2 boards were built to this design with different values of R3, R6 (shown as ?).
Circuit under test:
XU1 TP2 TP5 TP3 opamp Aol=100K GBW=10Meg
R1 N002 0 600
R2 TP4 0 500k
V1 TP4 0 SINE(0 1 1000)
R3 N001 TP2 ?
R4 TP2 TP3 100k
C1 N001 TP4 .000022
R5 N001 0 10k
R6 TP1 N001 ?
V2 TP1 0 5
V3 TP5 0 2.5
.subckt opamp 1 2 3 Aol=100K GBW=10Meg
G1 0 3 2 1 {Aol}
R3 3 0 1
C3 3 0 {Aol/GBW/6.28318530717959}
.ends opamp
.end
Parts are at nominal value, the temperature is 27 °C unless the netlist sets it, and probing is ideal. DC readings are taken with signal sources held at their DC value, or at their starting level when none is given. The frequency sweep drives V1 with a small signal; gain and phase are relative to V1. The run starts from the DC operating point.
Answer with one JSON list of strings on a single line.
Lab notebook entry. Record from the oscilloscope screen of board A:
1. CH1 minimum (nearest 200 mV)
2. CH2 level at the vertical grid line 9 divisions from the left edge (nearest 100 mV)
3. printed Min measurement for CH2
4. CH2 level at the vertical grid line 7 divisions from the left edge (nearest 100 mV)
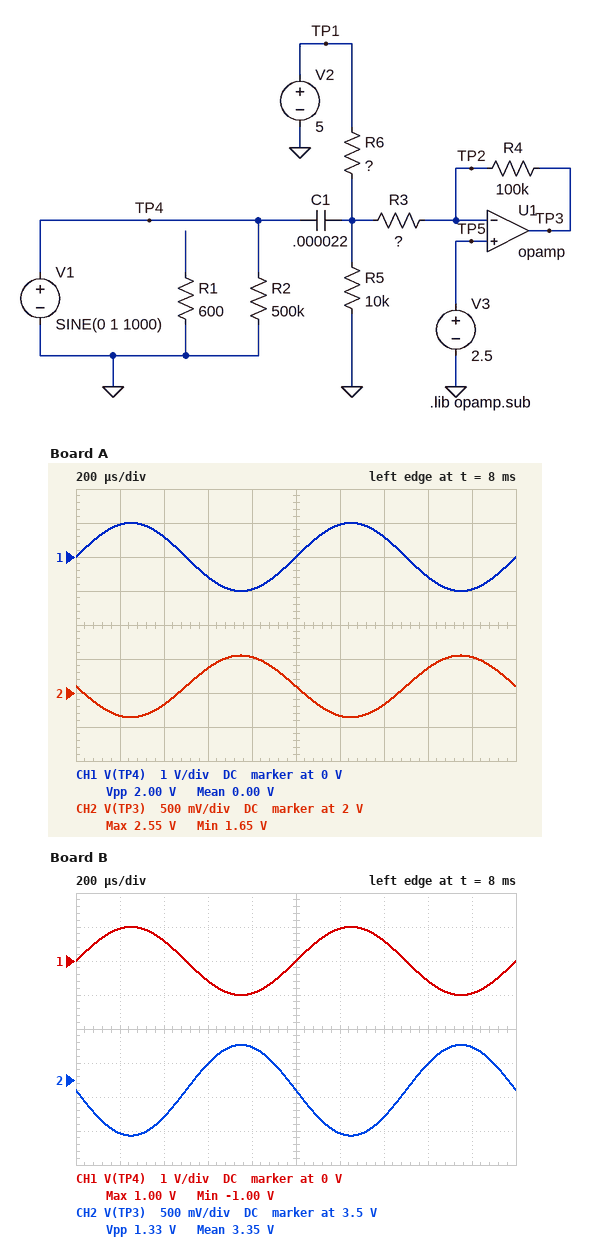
["-1.0 V", "2.5 V", "1.65 V", "1.8 V"]
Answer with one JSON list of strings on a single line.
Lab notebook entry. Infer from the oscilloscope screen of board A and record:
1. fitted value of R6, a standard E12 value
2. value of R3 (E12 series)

["4.7 kΩ", "220 kΩ"]
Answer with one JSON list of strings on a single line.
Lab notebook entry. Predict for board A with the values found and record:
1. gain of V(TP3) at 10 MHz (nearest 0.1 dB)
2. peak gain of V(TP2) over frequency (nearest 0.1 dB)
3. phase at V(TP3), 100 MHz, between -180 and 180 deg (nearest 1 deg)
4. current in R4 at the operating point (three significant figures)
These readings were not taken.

["-11.8 dB", "-10.1 dB", "94 deg", "4.04 µA"]
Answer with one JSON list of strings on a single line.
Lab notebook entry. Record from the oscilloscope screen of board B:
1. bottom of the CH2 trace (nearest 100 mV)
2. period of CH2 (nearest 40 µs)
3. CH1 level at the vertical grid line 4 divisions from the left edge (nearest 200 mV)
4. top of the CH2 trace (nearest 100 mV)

["2.7 V", "1.00 ms", "-1.0 V", "4.0 V"]
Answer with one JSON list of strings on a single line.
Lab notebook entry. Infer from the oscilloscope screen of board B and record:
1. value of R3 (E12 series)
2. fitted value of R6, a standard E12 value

["150 kΩ", "33 kΩ"]
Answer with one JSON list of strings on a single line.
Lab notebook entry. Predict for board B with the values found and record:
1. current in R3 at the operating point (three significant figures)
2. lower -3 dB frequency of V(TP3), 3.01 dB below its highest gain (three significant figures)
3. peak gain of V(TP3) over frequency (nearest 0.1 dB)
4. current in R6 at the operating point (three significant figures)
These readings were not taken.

["8.48 µA", "991 mHz", "-3.5 dB", "114 µA"]
